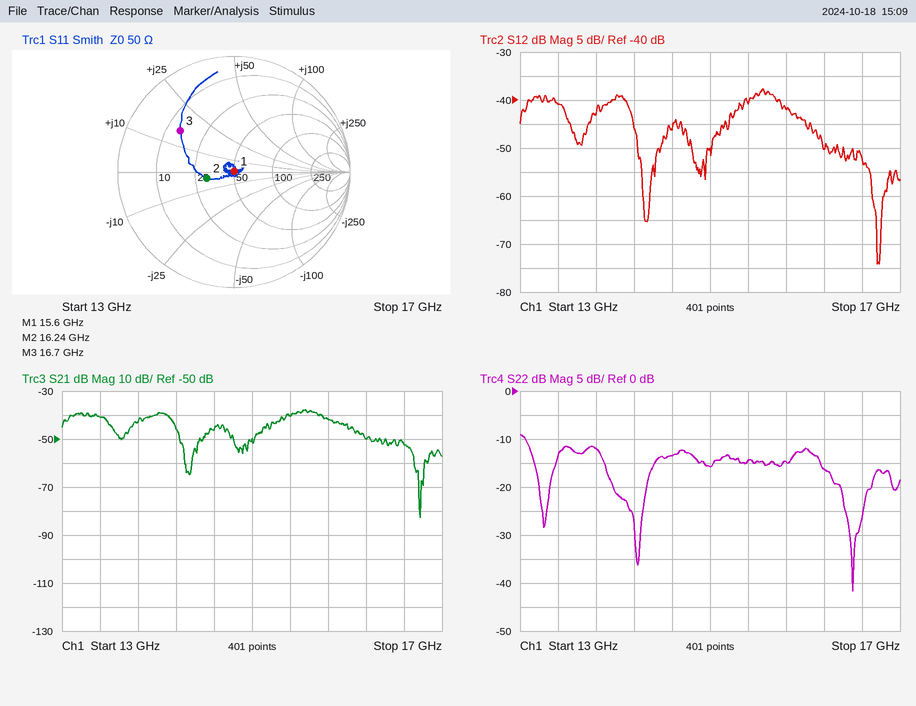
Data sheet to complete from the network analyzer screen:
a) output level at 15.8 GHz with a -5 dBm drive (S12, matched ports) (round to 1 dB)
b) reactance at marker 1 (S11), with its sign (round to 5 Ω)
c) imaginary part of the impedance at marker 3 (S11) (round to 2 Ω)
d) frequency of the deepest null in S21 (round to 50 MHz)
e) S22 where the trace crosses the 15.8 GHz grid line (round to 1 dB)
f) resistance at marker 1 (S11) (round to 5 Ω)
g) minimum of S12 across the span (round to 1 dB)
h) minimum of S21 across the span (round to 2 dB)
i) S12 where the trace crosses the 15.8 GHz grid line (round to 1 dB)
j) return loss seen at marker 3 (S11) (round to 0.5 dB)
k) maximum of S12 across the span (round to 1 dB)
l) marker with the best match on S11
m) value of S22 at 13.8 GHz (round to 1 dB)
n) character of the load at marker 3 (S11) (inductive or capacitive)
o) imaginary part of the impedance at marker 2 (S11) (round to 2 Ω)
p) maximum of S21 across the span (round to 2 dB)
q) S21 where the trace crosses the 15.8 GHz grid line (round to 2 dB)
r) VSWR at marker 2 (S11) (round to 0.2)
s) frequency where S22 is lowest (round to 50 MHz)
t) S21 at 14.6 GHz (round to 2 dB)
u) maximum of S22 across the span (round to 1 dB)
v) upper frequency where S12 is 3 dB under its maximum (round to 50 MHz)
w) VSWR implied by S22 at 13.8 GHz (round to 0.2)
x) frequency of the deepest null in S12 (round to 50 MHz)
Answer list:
-47 dBm
0 Ω
+16 Ω
16.75 GHz
-15 dB
50 Ω
-74 dB
-82 dB
-42 dB
4.5 dB
-38 dB
marker 1
-12 dB
inductive
-4 Ω
-38 dB
-42 dB
1.6
16.50 GHz
-46 dB
-9 dB
15.75 GHz
1.6
16.75 GHz
